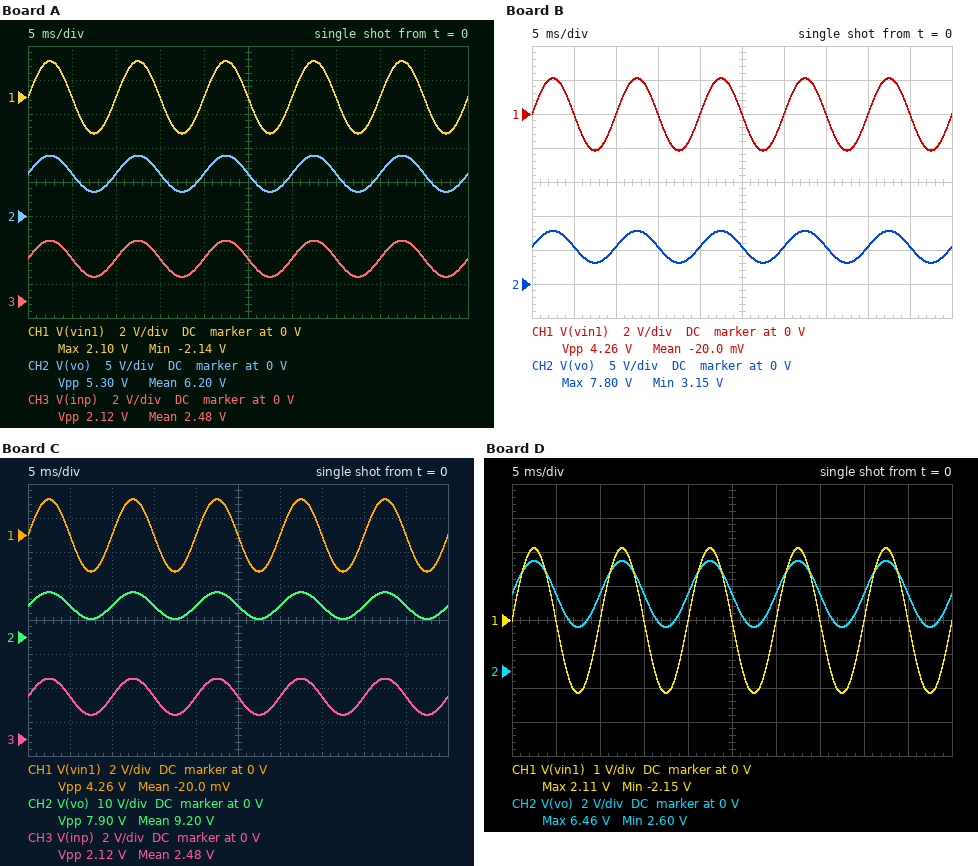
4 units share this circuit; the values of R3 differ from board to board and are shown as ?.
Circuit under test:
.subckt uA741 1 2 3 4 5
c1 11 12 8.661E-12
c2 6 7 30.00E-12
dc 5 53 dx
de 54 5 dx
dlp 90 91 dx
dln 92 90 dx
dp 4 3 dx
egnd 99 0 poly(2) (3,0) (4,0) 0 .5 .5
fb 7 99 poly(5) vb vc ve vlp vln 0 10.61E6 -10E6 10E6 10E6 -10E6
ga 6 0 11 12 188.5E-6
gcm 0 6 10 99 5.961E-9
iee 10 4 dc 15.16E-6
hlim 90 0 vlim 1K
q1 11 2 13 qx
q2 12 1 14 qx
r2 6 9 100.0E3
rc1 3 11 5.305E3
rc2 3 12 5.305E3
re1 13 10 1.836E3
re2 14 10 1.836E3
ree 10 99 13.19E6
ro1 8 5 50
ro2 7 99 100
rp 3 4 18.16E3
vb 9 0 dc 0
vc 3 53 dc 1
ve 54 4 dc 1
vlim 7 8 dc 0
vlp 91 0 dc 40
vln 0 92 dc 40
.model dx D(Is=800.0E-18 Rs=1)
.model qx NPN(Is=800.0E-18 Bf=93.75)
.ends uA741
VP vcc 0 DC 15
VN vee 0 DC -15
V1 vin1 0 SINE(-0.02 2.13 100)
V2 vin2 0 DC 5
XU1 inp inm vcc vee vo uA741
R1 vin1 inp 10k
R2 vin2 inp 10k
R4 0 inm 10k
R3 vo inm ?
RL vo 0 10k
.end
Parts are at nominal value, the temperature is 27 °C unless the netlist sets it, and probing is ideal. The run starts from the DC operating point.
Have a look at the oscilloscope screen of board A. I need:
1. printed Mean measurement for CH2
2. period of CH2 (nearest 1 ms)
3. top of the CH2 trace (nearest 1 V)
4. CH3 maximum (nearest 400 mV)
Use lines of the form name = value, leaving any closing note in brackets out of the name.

printed Mean measurement for CH2 = 6.20 V
period of CH2 = 10 ms
top of the CH2 trace = 9 V
CH3 maximum = 3.6 V
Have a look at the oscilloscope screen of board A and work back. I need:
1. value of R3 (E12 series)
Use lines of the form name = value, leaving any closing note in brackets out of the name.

value of R3 = 15 kΩ
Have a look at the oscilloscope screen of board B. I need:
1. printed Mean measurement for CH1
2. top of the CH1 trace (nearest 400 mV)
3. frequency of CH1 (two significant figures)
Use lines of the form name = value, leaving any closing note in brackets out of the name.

printed Mean measurement for CH1 = -20.0 mV
top of the CH1 trace = 2.0 V
frequency of CH1 = 100 Hz
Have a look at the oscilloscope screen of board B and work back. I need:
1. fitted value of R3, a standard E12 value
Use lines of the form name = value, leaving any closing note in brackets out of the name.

fitted value of R3, a standard E12 value = 12 kΩ
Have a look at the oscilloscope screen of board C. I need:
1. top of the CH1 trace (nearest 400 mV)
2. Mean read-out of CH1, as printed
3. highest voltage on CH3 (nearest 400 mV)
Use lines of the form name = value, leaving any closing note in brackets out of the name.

top of the CH1 trace = 2.0 V
Mean read-out of CH1, as printed = -20.0 mV
highest voltage on CH3 = 3.6 V
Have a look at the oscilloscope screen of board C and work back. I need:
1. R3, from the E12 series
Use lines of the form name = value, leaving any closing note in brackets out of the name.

R3, from the E12 series = 27 kΩ
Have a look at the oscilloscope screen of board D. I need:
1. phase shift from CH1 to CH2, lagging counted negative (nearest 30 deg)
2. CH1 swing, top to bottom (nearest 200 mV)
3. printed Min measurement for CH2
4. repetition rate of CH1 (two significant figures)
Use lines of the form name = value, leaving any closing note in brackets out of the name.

phase shift from CH1 to CH2, lagging counted negative = 0 deg
CH1 swing, top to bottom = 4.2 V
printed Min measurement for CH2 = 2.60 V
repetition rate of CH1 = 100 Hz
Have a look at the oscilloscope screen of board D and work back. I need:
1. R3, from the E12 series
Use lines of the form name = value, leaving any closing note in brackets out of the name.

R3, from the E12 series = 8.2 kΩ
